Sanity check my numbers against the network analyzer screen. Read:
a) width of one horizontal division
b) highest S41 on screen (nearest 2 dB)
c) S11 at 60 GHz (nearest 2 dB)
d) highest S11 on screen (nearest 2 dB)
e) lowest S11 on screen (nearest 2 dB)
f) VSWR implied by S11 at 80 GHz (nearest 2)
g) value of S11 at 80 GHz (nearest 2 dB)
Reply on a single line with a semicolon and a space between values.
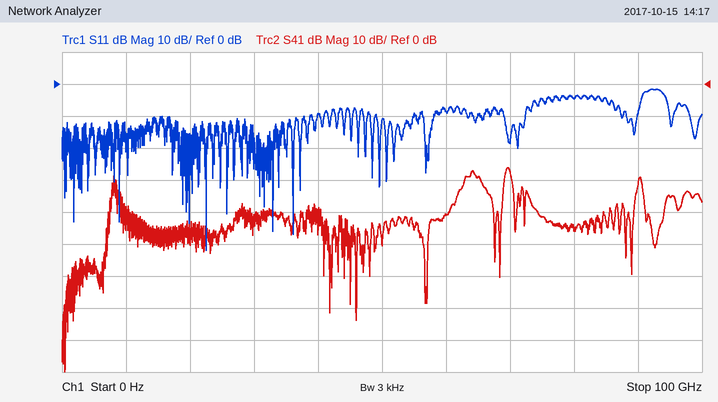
10 GHz; -26 dB; -8 dB; -2 dB; -52 dB; 4; -4 dB
